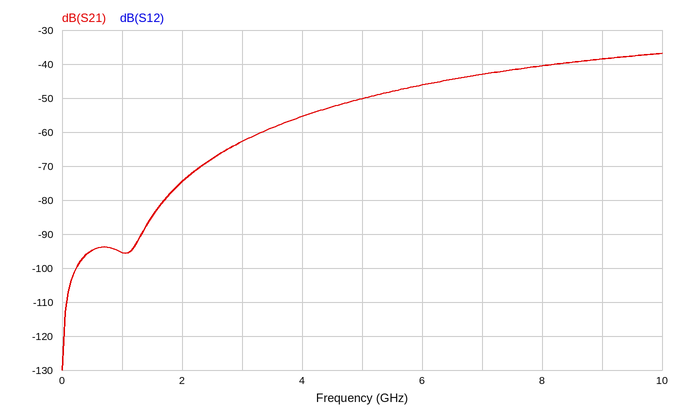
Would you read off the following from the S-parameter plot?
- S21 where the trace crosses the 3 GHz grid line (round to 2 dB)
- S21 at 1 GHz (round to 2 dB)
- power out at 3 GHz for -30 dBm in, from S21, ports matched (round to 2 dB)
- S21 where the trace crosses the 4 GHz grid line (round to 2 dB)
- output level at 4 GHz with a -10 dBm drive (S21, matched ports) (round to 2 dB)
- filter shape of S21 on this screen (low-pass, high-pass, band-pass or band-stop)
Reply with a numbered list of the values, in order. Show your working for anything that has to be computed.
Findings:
1. -62 dB
2. -96 dB
3. -30 dBm + (-62 dB) = -92 dBm
4. -56 dB
5. -10 dBm + (-56 dB) = -66 dBm
6. high-pass
